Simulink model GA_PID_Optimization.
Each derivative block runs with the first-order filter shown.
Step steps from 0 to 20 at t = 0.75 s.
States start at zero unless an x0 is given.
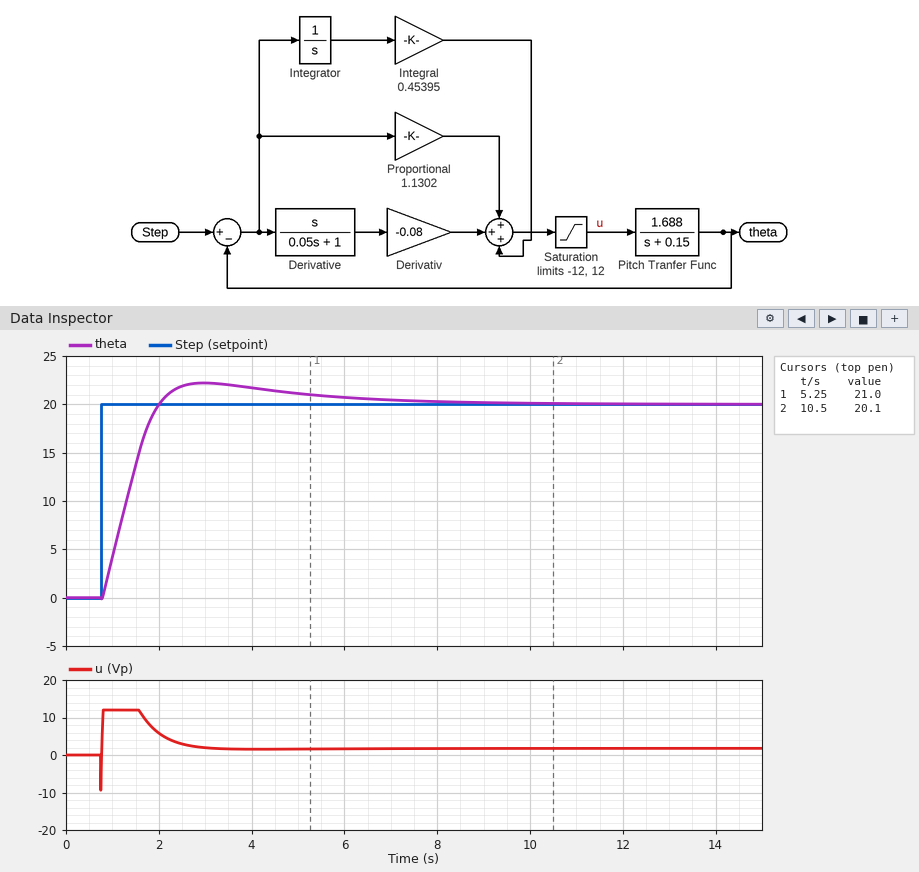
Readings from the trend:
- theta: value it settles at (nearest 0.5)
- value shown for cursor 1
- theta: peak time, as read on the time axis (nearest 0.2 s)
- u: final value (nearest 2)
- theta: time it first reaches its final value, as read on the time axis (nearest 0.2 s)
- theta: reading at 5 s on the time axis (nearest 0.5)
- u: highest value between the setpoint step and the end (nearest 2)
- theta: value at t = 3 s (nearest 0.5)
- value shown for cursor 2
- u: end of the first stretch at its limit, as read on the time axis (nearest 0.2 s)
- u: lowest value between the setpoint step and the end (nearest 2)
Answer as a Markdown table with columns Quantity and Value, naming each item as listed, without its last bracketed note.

| Quantity | Value |
|---|---|
| theta: value it settles at | 20.0 |
| value shown for cursor 1 | 21.0 |
| theta: peak time, as read on the time axis | 3.0 s |
| u: final value | 2 |
| theta: time it first reaches its final value, as read on the time axis | 2.0 s |
| theta: reading at 5 s on the time axis | 21.0 |
| u: highest value between the setpoint step and the end | 12 |
| theta: value at t = 3 s | 22.0 |
| value shown for cursor 2 | 20.1 |
| u: end of the first stretch at its limit, as read on the time axis | 1.6 s |
| u: lowest value between the setpoint step and the end | -10 |
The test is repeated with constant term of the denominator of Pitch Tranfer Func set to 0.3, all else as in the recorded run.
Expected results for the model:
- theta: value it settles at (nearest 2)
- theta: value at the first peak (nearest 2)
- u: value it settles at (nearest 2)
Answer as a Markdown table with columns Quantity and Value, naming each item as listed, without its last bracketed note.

| Quantity | Value |
|---|---|
| theta: value it settles at | 20 |
| theta: value at the first peak | 22 |
| u: value it settles at | 4 |
